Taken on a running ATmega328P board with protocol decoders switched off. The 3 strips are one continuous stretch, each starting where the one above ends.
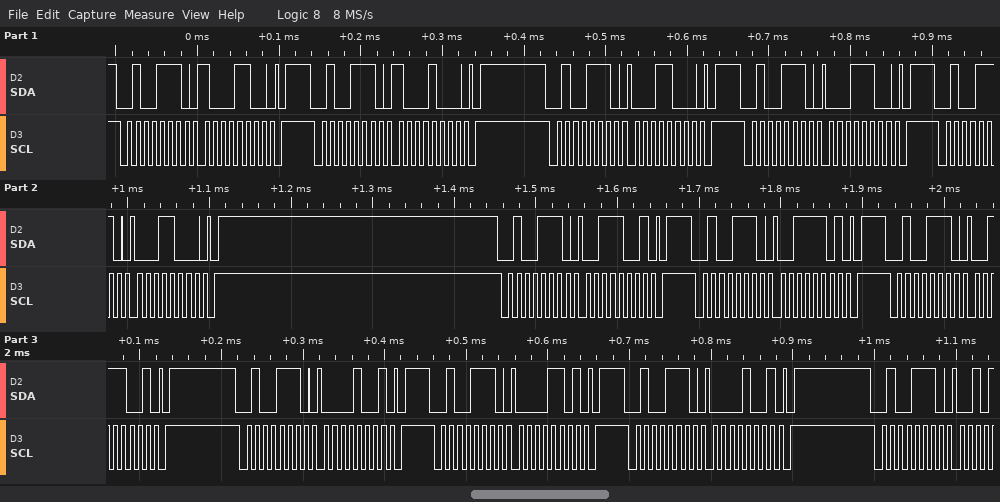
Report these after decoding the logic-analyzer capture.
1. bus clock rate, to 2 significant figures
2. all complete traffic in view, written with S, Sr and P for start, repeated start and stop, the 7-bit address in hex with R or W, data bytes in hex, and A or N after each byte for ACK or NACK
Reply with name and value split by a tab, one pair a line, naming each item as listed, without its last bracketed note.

bus clock rate, to 2 significant figures	100 kHz
all complete traffic in view, written with S, Sr and P for start, repeated start and stop, the 7-bit address in hex with R or W, data bytes in hex, and A or N after each byte for ACK or NACK	S 27W A 8C A P S 27W A 88 A P S 27W A 18 A P S 27W A 1C A P S 27W A 18 A P S 27W A 39 A P S 27W A 3D A P S 27W A 39 A P S 27W A 09 A P S 27W A 0D A P S 27W A 09 A P S 27W A
